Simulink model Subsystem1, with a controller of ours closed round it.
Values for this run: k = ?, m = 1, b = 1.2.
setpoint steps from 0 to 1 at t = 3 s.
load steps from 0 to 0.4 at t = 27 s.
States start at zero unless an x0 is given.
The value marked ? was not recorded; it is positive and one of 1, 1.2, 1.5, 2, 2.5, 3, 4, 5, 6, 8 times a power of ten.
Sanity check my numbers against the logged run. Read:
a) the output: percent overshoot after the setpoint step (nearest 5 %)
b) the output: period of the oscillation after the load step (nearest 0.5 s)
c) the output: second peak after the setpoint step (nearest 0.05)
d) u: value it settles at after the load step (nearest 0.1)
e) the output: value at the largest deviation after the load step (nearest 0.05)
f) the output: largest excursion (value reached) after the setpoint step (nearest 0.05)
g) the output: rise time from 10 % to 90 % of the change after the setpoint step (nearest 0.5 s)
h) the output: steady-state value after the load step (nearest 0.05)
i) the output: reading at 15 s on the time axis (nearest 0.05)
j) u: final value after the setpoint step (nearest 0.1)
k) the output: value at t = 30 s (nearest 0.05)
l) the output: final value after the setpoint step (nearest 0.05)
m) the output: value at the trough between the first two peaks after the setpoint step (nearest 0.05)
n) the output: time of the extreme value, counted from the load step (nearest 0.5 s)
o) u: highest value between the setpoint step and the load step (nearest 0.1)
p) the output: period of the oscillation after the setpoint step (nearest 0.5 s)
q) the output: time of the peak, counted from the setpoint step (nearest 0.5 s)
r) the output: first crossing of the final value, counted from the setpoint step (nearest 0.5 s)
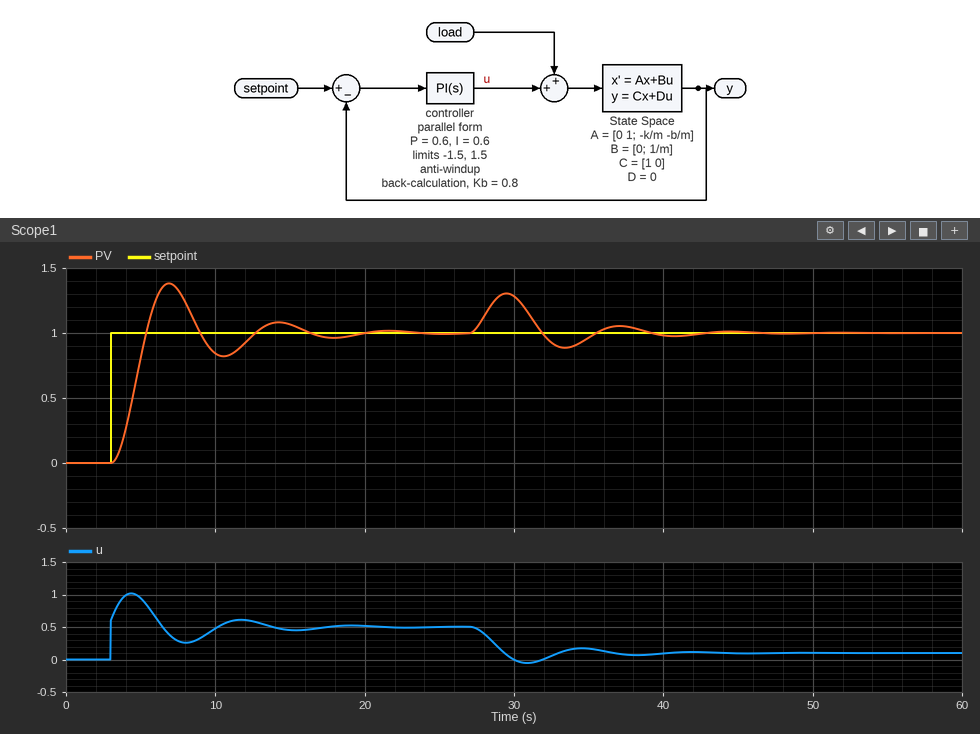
40 %
7.5 s
1.10
0.1
1.30
1.40
1.5 s
1.00
1.05
0.5
1.30
1.00
0.80
2.5 s
1.0
7.5 s
4.0 s
2.5 s
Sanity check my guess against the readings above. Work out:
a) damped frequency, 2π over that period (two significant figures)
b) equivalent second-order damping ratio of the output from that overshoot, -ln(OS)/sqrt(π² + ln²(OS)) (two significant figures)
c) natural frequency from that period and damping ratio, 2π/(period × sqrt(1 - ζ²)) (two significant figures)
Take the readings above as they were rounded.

0.84 rad/s
0.28
0.87 rad/s
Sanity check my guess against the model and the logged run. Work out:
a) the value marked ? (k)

0.5
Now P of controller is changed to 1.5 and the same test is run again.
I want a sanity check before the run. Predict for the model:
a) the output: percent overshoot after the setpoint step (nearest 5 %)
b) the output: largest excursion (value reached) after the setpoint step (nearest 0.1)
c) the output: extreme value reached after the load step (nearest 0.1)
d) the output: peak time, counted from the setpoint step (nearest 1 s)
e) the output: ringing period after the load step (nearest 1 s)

25 %
1.2
1.2
3 s
5 s
